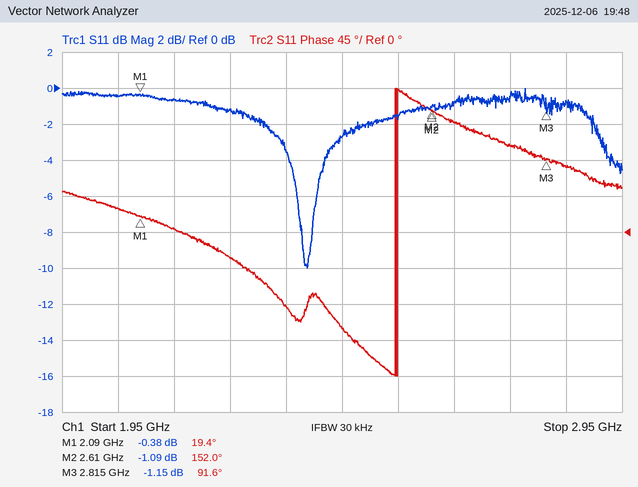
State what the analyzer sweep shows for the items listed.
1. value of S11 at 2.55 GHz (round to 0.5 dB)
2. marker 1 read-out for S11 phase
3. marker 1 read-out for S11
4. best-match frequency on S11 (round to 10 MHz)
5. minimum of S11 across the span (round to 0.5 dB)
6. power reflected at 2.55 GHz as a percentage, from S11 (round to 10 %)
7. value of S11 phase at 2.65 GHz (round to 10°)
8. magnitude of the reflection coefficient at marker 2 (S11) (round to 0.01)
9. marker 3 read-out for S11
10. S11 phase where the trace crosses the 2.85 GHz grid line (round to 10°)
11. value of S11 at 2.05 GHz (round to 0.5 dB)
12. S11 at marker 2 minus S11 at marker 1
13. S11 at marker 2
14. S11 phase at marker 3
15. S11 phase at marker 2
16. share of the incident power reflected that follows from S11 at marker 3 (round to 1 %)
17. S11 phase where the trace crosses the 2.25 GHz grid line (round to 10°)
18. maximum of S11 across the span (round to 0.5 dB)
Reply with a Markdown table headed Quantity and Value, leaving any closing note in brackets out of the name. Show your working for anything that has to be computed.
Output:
| Quantity | Value |
|---|---|
| value of S11 at 2.55 GHz | -1.5 dB |
| marker 1 read-out for S11 phase | 19.4° |
| marker 1 read-out for S11 | -0.38 dB |
| best-match frequency on S11 | 2.39 GHz |
| minimum of S11 across the span | -10.0 dB |
| power reflected at 2.55 GHz as a percentage, from S11 | 10^(-1.5/10) ≈ 70.8 %, so 70 % to the nearest 10 % |
| value of S11 phase at 2.65 GHz | 140° |
| magnitude of the reflection coefficient at marker 2 (S11) | 10^(-1.09/20) ≈ 0.88 |
| marker 3 read-out for S11 | -1.15 dB |
| S11 phase where the trace crosses the 2.85 GHz grid line | 80° |
| value of S11 at 2.05 GHz | -0.5 dB |
| S11 at marker 2 minus S11 at marker 1 | -1.09 − (-0.38) = -0.71 dB |
| S11 at marker 2 | -1.09 dB |
| S11 phase at marker 3 | 91.6° |
| S11 phase at marker 2 | 152.0° |
| share of the incident power reflected that follows from S11 at marker 3 | 10^(-1.15/10) ≈ 77 % |
| S11 phase where the trace crosses the 2.25 GHz grid line | -30° |
| maximum of S11 across the span | 0.0 dB |
